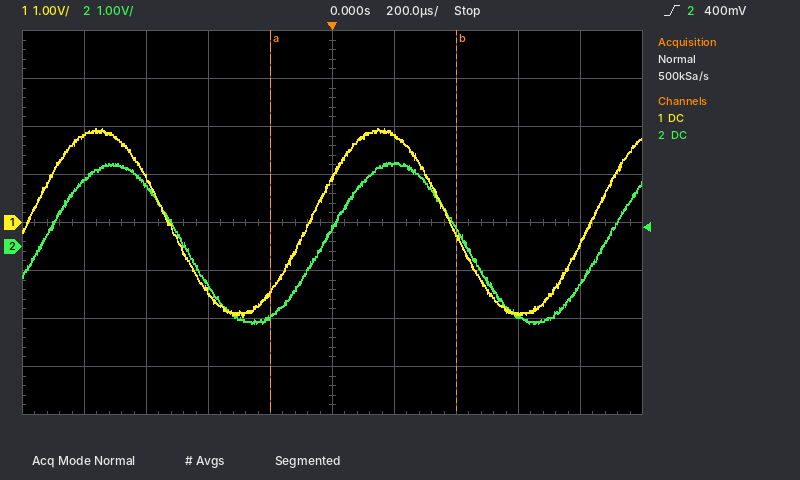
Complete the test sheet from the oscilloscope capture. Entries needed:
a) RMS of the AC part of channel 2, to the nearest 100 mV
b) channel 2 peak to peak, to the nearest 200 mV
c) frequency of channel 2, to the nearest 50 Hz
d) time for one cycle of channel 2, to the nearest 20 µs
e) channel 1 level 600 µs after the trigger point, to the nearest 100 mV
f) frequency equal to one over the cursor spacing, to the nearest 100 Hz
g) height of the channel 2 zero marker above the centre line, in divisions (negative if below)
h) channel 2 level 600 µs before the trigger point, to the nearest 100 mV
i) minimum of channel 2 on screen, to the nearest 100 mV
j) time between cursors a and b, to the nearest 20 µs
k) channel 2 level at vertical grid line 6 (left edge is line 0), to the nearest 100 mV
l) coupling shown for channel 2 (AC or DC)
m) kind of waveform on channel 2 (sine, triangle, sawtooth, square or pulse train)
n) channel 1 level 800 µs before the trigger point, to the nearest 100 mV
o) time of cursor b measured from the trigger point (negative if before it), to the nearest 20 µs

1.2 V
3.4 V
1.10 kHz
900 µs
-1.9 V
1.7 kHz
-0.5 div
1.3 V
-1.6 V
600 µs
1.7 V
DC
sine
1.8 V
+400 µs
